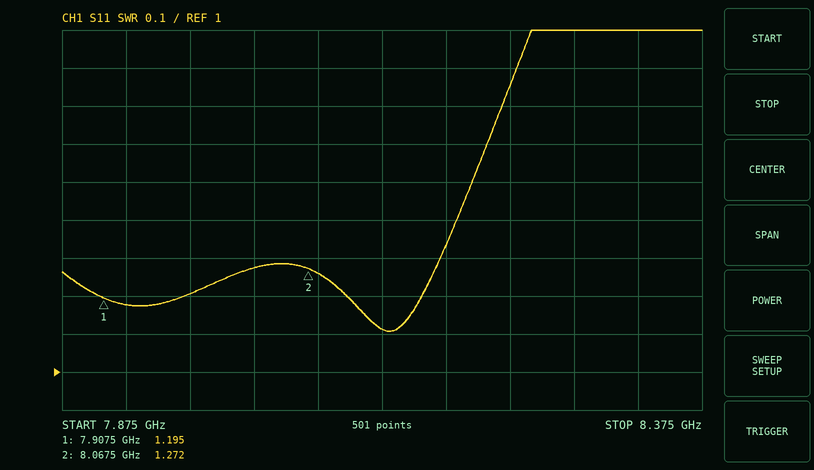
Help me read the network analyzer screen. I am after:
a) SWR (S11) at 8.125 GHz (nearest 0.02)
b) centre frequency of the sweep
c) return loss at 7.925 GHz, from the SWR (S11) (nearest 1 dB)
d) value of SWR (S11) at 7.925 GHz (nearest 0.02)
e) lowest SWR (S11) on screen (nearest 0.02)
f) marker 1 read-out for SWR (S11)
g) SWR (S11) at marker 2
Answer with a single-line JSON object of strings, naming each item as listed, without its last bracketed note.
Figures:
{"SWR (S11) at 8.125 GHz": "1.12", "centre frequency of the sweep": "8.125 GHz", "return loss at 7.925 GHz, from the SWR (S11)": "22 dB", "value of SWR (S11) at 7.925 GHz": "1.18", "lowest SWR (S11) on screen": "1.10", "marker 1 read-out for SWR": "1.195", "SWR (S11) at marker 2": "1.272"}
